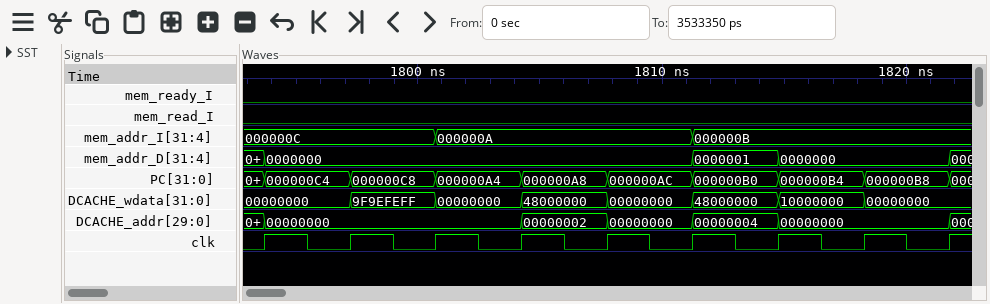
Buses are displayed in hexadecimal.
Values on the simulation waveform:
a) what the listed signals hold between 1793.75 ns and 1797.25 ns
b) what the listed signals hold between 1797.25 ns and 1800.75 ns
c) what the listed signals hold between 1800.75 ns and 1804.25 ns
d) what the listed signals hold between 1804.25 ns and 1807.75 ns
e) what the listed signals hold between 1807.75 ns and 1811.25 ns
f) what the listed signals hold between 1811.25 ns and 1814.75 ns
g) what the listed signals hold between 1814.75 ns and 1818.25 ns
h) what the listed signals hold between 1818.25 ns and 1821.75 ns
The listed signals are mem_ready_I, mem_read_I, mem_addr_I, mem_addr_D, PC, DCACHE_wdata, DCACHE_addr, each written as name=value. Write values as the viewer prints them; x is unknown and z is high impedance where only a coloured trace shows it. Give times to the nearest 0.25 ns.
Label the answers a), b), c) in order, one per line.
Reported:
a) mem_ready_I=0, mem_read_I=0, mem_addr_I=000000C, mem_addr_D=0000000, PC=000000C4, DCACHE_wdata=00000000, DCACHE_addr=00000000
b) mem_ready_I=0, mem_read_I=0, mem_addr_I=000000C, mem_addr_D=0000000, PC=000000C8, DCACHE_wdata=9F9EFEFF, DCACHE_addr=00000000
c) mem_ready_I=0, mem_read_I=0, mem_addr_I=000000A, mem_addr_D=0000000, PC=000000A4, DCACHE_wdata=00000000, DCACHE_addr=00000000
d) mem_ready_I=0, mem_read_I=0, mem_addr_I=000000A, mem_addr_D=0000000, PC=000000A8, DCACHE_wdata=48000000, DCACHE_addr=00000002
e) mem_ready_I=0, mem_read_I=0, mem_addr_I=000000A, mem_addr_D=0000000, PC=000000AC, DCACHE_wdata=00000000, DCACHE_addr=00000000
f) mem_ready_I=0, mem_read_I=0, mem_addr_I=000000B, mem_addr_D=0000001, PC=000000B0, DCACHE_wdata=48000000, DCACHE_addr=00000004
g) mem_ready_I=0, mem_read_I=0, mem_addr_I=000000B, mem_addr_D=0000000, PC=000000B4, DCACHE_wdata=10000000, DCACHE_addr=00000000
h) mem_ready_I=0, mem_read_I=0, mem_addr_I=000000B, mem_addr_D=0000000, PC=000000B8, DCACHE_wdata=00000000, DCACHE_addr=00000000
